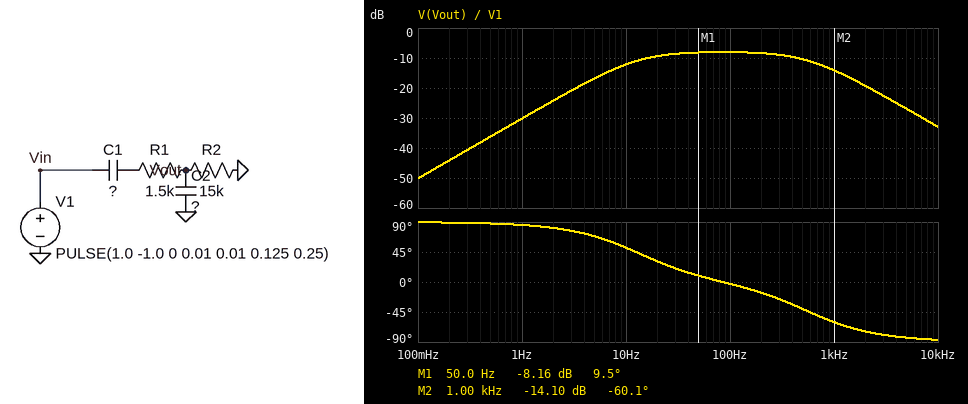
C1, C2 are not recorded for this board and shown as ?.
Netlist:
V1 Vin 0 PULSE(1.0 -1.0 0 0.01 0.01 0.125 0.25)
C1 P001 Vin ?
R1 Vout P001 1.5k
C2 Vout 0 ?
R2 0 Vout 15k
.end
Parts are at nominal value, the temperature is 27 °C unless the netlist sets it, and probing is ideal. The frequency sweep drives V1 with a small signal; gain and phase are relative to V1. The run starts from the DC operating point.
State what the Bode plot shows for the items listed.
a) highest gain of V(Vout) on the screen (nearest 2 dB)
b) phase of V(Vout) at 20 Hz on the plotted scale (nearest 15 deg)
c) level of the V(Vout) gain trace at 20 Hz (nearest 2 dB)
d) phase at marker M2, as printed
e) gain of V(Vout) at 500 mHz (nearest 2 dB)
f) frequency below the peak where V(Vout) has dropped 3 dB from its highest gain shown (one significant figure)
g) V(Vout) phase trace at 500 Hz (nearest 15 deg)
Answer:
-8 dB
30 deg
-10 dB
-60.1 deg
-36 dB
10 Hz
-45 deg
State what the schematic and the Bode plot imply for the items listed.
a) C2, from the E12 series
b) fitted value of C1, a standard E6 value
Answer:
470 nF
330 nF
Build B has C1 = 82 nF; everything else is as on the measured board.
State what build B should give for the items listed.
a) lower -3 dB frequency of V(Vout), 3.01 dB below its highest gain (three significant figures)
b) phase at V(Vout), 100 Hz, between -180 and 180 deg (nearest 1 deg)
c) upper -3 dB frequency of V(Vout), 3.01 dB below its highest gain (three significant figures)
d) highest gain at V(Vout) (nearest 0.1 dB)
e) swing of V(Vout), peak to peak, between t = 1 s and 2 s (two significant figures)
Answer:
18.7 Hz
7 deg
1.56 kHz
-16.7 dB
340 mV
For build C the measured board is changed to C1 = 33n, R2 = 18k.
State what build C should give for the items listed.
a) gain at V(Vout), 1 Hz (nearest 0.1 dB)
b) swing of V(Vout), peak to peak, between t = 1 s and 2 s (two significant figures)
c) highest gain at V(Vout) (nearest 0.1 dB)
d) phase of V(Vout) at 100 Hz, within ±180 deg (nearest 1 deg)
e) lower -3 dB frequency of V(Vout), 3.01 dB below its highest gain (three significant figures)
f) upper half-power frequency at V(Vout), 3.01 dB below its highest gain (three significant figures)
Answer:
-48.6 dB
160 mV
-23.7 dB
8 deg
17.4 Hz
3.48 kHz
